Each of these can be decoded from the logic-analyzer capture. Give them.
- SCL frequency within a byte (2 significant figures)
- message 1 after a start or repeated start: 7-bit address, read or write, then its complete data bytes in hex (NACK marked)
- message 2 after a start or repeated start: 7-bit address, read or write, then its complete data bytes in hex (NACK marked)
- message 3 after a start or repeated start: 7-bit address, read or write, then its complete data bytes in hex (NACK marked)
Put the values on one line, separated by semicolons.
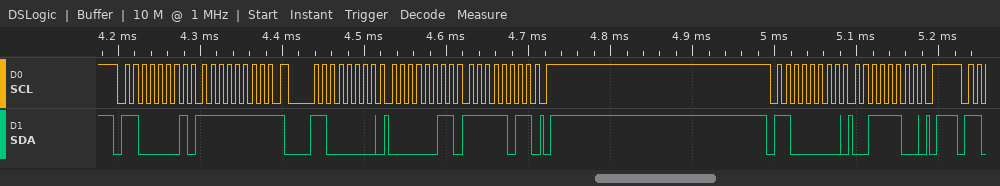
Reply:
100 kHz; 0x60 read: FF NACK; 0x60 write: 03 FB; 0x60 write: 3C
